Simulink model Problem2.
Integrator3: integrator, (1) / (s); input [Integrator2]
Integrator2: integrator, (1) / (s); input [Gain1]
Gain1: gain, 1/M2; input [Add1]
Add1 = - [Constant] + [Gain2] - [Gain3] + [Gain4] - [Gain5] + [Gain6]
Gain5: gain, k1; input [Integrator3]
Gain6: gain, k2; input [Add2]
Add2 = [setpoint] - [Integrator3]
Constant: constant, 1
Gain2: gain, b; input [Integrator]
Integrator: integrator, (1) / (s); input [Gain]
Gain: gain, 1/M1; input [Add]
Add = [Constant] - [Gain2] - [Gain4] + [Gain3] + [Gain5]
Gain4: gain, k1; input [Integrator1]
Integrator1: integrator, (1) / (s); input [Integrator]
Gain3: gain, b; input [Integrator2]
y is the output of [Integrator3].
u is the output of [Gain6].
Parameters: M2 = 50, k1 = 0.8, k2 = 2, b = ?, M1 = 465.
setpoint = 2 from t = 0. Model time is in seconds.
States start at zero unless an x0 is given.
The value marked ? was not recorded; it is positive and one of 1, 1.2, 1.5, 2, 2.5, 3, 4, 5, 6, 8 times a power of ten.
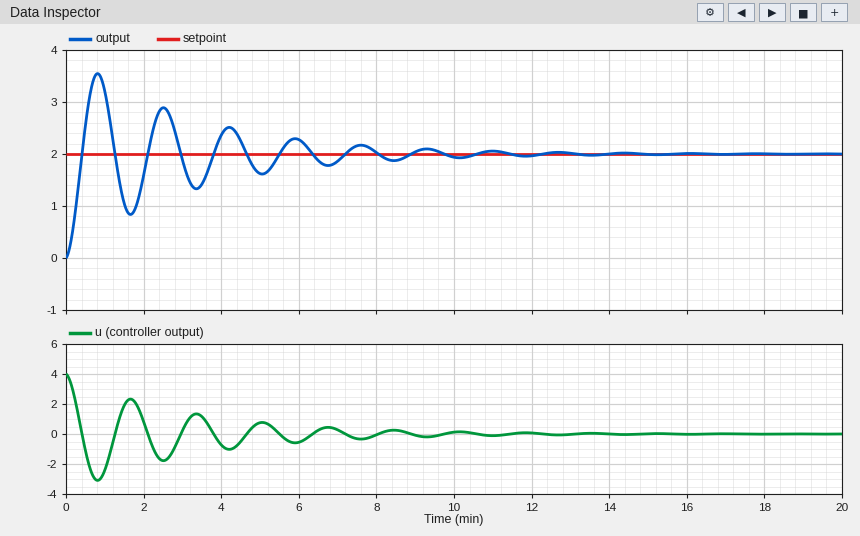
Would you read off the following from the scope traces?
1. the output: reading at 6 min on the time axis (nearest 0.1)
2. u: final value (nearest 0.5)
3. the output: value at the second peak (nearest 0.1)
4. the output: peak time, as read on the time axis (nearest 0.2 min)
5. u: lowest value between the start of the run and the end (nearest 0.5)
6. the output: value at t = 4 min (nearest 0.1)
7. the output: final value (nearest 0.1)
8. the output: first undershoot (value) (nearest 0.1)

2.3
0.0
2.9
0.8 min
-3.0
2.4
2.0
0.8
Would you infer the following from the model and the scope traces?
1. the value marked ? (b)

150
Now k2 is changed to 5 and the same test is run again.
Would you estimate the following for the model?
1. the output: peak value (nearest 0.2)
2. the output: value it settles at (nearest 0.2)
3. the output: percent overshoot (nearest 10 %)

3.4
2.0
70 %
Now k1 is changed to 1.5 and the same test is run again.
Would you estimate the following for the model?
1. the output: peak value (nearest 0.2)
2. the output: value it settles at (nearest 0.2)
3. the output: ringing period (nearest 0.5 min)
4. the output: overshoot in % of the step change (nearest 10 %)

3.6
2.0
1.5 min
80 %
